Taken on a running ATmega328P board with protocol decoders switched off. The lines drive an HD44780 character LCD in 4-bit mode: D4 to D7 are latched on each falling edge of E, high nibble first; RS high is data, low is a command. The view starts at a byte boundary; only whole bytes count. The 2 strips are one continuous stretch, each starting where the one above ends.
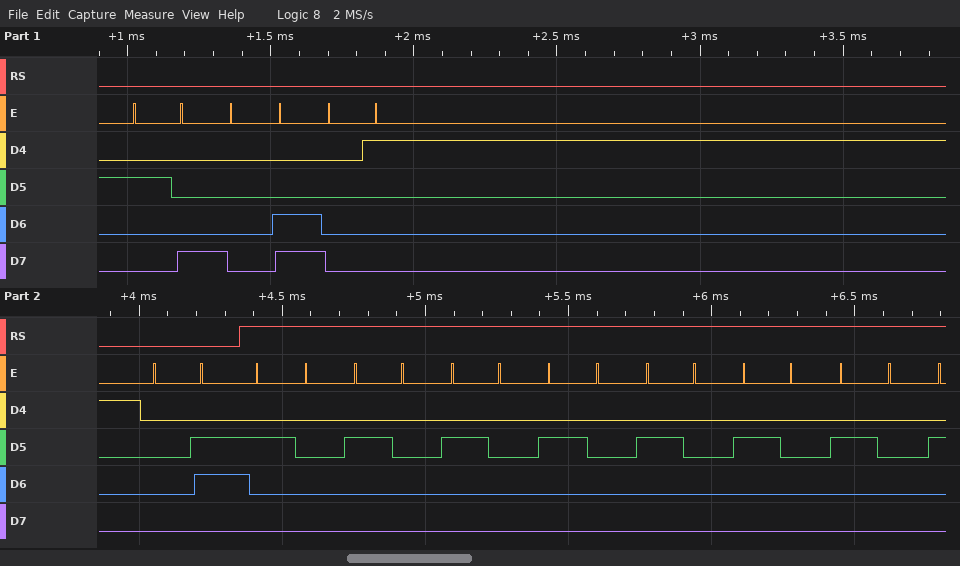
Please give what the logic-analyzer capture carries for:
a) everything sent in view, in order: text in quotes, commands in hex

0x28 0x0C 0x01 0x06 "       "
